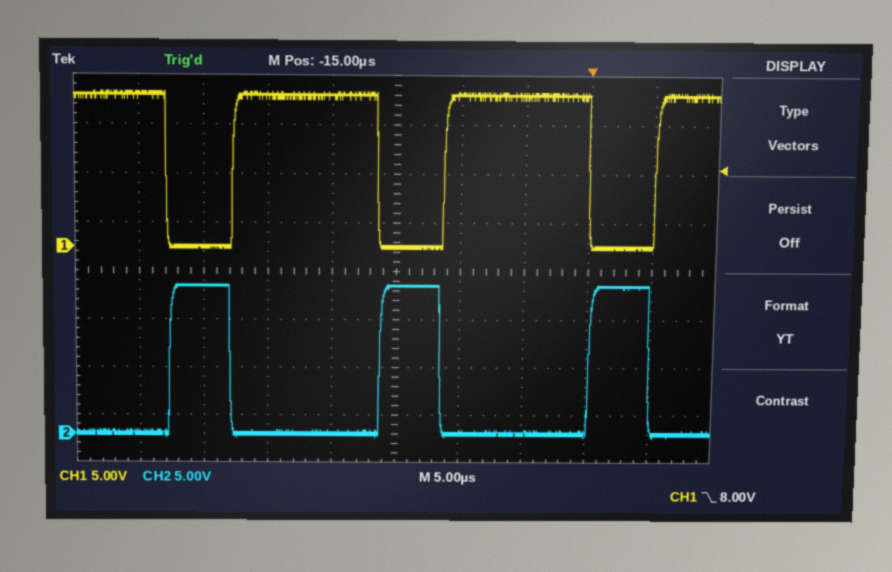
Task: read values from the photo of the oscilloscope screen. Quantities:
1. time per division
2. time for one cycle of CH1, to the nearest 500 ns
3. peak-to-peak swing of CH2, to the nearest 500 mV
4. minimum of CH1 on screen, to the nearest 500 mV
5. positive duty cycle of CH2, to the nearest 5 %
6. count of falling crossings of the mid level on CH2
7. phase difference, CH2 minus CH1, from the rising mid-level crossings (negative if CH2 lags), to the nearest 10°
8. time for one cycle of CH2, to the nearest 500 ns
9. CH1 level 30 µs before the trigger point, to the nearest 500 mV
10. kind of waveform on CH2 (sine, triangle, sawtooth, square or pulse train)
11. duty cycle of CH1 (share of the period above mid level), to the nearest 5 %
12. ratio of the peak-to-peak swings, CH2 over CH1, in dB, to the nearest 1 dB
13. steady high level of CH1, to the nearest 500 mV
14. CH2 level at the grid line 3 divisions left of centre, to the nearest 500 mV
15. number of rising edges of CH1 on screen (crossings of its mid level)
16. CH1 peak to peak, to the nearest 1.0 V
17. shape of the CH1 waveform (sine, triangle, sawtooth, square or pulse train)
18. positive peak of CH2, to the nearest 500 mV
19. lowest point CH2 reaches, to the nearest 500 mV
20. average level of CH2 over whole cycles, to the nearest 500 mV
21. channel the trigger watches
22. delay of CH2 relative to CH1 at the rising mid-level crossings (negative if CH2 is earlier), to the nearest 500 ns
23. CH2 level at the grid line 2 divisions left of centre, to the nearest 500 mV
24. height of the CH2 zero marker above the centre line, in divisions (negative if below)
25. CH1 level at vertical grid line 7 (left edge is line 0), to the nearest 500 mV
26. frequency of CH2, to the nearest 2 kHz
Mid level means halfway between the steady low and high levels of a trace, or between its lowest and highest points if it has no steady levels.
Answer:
5 µs
16.5 µs
16.0 V
0.0 V
30 %
3
+110°
16.5 µs
0.0 V
pulse train
70 %
0 dB
15.5 V
15.5 V
3
16.0 V
pulse train
15.5 V
-500 mV
4.5 V
CH1
-5.0 µs
0.0 V
-3.4 div
15.5 V
60 kHz
